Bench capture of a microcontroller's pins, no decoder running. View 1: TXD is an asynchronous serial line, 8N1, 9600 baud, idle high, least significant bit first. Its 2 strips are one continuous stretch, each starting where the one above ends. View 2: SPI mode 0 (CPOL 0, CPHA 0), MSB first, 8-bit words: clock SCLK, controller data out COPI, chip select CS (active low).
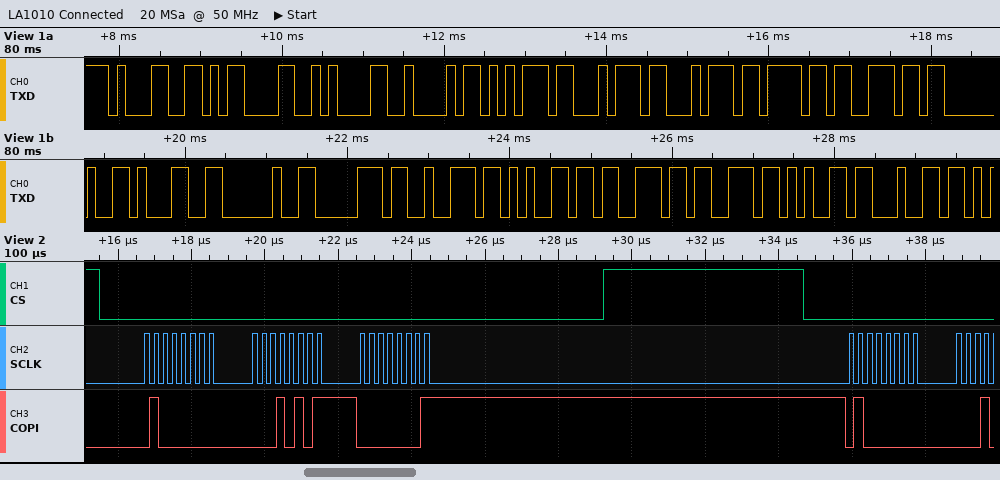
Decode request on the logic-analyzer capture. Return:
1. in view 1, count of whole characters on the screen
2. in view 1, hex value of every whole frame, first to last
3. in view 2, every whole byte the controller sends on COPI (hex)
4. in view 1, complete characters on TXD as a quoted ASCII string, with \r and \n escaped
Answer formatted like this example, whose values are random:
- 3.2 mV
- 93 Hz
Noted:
- 19
- 31 0D 0A 42 75 74 74 6F 6E 20 31 20 70 72 65 73 73 65 64
- 0x40 0x15 0x01 0x40
- "1\r\nButton 1 pressed"
